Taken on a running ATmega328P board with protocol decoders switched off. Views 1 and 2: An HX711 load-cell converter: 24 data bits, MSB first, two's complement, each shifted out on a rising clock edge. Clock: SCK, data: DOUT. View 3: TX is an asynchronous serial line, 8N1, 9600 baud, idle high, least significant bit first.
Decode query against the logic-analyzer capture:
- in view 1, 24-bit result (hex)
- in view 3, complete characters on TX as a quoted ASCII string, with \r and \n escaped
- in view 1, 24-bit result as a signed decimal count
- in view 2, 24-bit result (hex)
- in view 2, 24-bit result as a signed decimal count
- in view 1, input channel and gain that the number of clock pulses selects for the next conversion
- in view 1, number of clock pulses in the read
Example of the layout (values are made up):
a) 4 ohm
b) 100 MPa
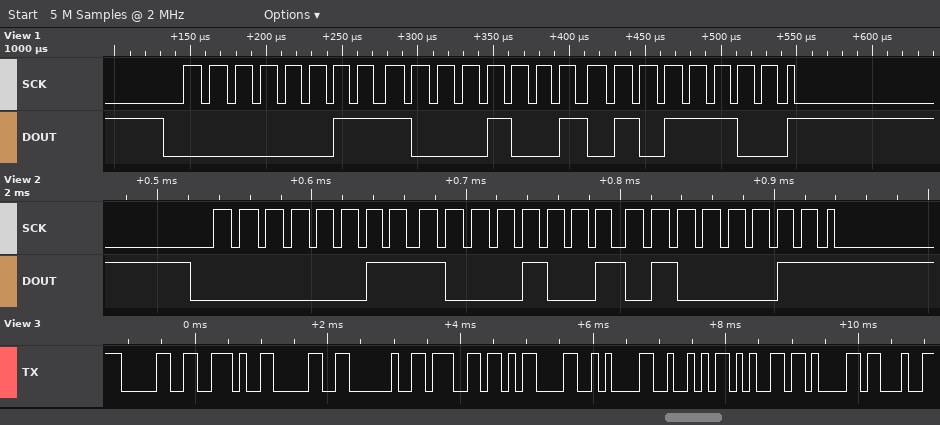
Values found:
a) 0x03895C
b) "0.0 g\r\nRea"
c) 231772
d) 0x038943
e) 231747
f) channel A, gain 128
g) 25
